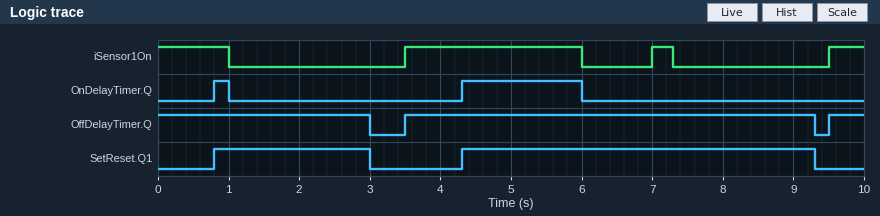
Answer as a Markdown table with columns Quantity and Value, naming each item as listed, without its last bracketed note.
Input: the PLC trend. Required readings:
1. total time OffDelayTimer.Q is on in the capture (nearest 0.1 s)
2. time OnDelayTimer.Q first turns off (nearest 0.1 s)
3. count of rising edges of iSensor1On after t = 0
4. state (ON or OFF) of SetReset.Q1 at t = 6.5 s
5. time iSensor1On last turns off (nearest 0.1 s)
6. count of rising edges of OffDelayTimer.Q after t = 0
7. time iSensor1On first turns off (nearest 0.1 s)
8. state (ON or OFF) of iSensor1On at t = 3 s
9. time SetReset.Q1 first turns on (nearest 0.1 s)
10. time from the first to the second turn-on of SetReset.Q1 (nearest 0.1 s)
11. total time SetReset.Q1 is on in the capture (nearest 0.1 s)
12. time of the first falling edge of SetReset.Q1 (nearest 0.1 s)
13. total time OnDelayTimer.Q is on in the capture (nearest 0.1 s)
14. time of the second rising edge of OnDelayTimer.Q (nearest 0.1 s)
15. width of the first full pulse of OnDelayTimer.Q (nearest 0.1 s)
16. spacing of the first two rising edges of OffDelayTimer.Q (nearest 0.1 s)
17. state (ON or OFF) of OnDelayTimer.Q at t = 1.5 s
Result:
| Quantity | Value |
|---|---|
| total time OffDelayTimer.Q is on in the capture | 9.3 s |
| time OnDelayTimer.Q first turns off | 1.0 s |
| count of rising edges of iSensor1On after t = 0 | 3 |
| state (ON or OFF) of SetReset.Q1 at t = 6.5 s | ON |
| time iSensor1On last turns off | 7.3 s |
| count of rising edges of OffDelayTimer.Q after t = 0 | 2 |
| time iSensor1On first turns off | 1.0 s |
| state (ON or OFF) of iSensor1On at t = 3 s | OFF |
| time SetReset.Q1 first turns on | 0.8 s |
| time from the first to the second turn-on of SetReset.Q1 | 3.5 s |
| total time SetReset.Q1 is on in the capture | 7.2 s |
| time of the first falling edge of SetReset.Q1 | 3.0 s |
| total time OnDelayTimer.Q is on in the capture | 1.9 s |
| time of the second rising edge of OnDelayTimer.Q | 4.3 s |
| width of the first full pulse of OnDelayTimer.Q | 0.2 s |
| spacing of the first two rising edges of OffDelayTimer.Q | 6.0 s |
| state (ON or OFF) of OnDelayTimer.Q at t = 1.5 s | OFF |
